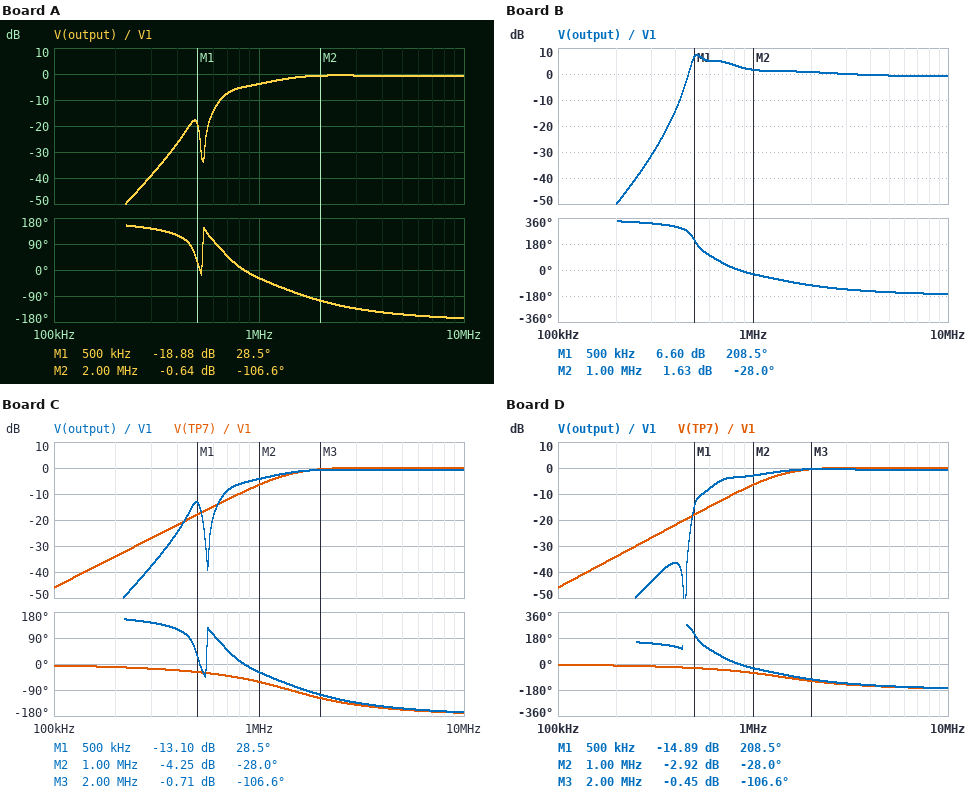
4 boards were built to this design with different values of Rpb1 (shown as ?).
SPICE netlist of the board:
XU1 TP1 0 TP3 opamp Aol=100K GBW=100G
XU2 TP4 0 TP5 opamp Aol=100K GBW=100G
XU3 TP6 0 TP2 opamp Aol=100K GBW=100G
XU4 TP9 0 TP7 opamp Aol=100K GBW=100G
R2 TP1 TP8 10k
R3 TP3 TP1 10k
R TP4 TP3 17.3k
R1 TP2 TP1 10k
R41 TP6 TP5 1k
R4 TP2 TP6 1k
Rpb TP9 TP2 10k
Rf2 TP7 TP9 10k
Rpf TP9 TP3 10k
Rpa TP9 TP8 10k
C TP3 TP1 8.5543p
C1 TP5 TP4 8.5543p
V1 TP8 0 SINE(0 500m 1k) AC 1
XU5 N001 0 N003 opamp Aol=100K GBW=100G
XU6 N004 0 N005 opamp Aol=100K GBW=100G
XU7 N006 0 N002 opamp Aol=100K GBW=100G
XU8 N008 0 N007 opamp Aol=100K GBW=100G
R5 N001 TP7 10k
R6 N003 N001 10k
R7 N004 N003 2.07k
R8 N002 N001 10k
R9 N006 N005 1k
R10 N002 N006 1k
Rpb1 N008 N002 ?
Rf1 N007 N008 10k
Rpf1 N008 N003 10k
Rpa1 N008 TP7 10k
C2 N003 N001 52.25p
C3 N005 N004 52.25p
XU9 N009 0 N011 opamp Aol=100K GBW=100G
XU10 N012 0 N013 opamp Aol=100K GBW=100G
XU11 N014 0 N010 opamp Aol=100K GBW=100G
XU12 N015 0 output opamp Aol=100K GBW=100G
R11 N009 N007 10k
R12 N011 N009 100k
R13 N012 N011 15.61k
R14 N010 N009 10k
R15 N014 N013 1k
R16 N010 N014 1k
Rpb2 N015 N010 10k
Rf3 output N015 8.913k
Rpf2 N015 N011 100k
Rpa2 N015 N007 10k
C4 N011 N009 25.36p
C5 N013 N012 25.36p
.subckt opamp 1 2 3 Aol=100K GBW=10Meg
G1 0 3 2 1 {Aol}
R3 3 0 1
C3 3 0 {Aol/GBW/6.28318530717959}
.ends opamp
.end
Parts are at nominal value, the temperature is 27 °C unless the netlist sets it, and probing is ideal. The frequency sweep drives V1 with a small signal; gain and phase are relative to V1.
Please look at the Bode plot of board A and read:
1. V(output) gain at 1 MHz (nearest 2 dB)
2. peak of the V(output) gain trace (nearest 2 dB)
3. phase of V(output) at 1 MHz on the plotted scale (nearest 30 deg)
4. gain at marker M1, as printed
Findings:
-4 dB
0 dB
-30 deg
-18.88 dB
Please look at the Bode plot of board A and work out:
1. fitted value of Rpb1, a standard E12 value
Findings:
27 kΩ
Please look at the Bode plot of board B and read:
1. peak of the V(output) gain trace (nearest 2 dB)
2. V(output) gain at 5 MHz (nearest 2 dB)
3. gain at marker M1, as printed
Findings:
8 dB
0 dB
6.60 dB
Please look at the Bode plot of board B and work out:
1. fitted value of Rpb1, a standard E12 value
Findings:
5.6 kΩ
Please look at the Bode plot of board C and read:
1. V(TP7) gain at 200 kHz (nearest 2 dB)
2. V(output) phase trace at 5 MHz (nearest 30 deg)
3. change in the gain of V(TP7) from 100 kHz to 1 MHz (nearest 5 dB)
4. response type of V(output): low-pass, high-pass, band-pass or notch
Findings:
-34 dB
-150 deg
40 dB
high-pass
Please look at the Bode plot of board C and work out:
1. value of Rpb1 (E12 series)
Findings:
33 kΩ
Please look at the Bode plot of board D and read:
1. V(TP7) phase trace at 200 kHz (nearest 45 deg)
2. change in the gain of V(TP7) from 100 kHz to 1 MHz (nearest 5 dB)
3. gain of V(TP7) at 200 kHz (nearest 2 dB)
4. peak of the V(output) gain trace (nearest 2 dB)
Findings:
0 deg
40 dB
-34 dB
0 dB
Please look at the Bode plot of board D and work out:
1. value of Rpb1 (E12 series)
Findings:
18 kΩ
